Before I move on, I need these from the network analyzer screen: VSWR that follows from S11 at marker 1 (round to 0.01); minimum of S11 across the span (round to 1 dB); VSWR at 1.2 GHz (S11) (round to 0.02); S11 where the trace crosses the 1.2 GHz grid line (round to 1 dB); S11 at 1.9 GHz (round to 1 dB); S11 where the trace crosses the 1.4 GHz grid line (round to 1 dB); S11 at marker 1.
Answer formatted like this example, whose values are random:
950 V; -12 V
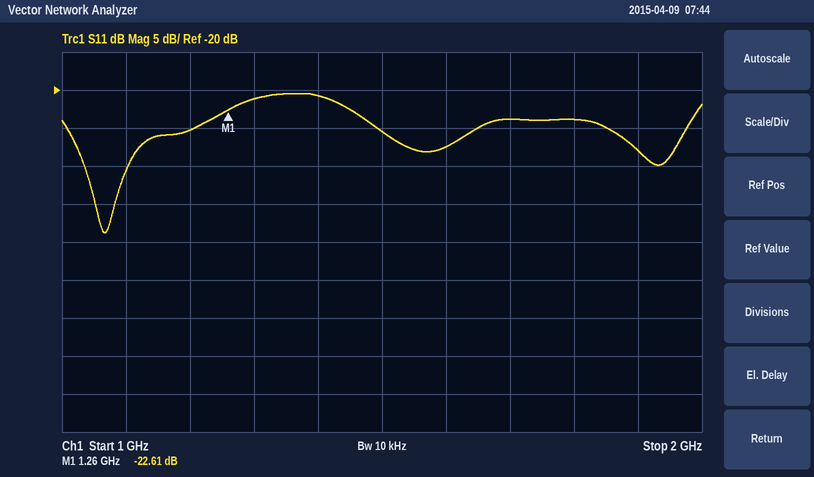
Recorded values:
1.16; -39 dB; 1.12; -25 dB; -28 dB; -21 dB; -22.61 dB
